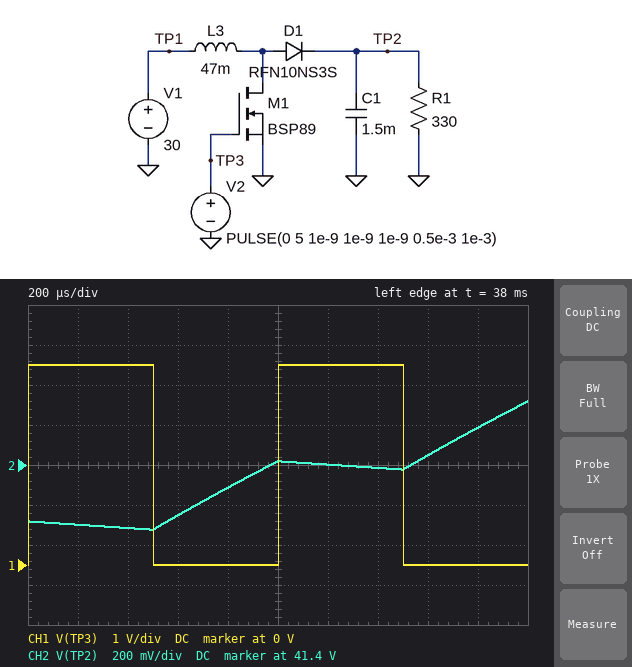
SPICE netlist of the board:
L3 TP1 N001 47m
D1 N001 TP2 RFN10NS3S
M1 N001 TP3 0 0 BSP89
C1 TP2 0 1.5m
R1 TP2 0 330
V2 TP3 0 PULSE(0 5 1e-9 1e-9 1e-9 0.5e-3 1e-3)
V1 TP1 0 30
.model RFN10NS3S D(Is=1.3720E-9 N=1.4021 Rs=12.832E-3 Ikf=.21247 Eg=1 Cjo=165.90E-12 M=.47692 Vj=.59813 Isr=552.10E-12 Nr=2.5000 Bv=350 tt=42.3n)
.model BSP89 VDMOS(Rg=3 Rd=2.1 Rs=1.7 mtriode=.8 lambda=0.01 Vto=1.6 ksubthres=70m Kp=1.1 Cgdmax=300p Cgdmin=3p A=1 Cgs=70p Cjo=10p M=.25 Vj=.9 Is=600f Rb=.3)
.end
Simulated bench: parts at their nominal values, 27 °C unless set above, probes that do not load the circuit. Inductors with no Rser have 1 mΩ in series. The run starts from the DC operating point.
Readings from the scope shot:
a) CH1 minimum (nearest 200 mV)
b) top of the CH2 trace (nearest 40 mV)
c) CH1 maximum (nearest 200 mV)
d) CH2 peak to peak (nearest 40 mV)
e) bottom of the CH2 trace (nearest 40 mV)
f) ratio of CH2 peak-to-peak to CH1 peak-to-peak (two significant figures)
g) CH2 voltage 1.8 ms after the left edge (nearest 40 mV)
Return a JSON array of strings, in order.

["0 V", "41.72 V", "5.0 V", "640 mV", "41.08 V", "0.13", "41.60 V"]
